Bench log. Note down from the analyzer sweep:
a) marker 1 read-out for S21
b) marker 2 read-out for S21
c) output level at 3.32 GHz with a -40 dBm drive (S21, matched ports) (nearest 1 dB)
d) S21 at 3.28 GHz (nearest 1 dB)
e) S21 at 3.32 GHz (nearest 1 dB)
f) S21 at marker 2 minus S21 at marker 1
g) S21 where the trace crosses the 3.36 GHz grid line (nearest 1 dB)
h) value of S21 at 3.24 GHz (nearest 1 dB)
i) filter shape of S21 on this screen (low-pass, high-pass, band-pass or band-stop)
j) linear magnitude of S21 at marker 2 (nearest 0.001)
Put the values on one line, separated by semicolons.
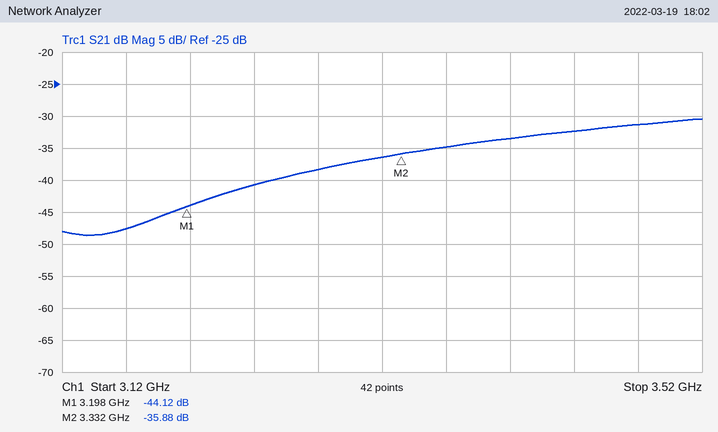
-44.12 dB; -35.88 dB; -76 dBm; -38 dB; -36 dB; 8.24 dB; -35 dB; -41 dB; high-pass; 0.016
